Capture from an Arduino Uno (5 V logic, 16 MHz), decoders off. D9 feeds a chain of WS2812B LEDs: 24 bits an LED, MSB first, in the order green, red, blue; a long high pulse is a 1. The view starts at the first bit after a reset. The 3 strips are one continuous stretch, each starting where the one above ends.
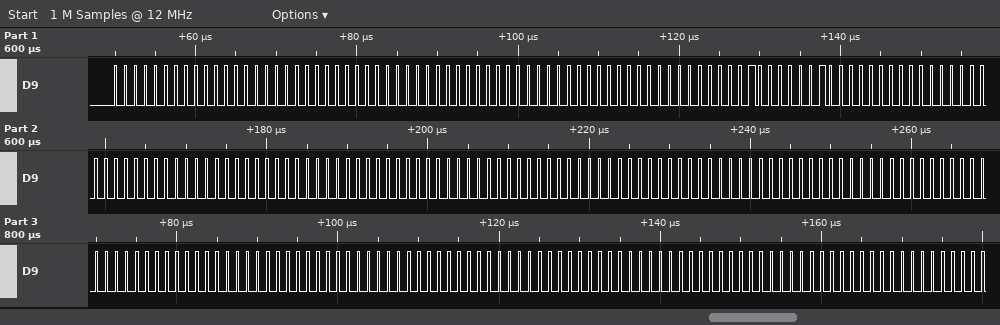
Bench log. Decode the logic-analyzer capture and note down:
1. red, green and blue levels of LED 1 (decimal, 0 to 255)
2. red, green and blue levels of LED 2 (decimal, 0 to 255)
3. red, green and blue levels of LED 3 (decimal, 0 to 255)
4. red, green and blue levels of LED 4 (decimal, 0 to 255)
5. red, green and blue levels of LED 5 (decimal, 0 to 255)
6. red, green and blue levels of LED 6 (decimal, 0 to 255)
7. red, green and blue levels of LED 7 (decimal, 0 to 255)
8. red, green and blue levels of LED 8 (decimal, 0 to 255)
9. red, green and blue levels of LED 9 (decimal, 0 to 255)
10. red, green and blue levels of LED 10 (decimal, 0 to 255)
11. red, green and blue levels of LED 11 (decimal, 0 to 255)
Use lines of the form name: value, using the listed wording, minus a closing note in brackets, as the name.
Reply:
red, green and blue levels of LED 1: 0, 0, 0
red, green and blue levels of LED 2: 0, 0, 0
red, green and blue levels of LED 3: 1, 0, 2
red, green and blue levels of LED 4: 0, 0, 0
red, green and blue levels of LED 5: 0, 0, 0
red, green and blue levels of LED 6: 0, 0, 0
red, green and blue levels of LED 7: 0, 0, 0
red, green and blue levels of LED 8: 0, 0, 0
red, green and blue levels of LED 9: 0, 0, 0
red, green and blue levels of LED 10: 0, 0, 0
red, green and blue levels of LED 11: 0, 0, 0
